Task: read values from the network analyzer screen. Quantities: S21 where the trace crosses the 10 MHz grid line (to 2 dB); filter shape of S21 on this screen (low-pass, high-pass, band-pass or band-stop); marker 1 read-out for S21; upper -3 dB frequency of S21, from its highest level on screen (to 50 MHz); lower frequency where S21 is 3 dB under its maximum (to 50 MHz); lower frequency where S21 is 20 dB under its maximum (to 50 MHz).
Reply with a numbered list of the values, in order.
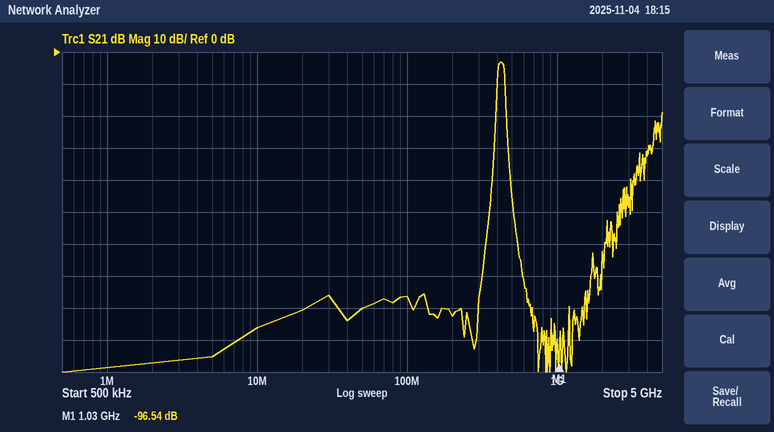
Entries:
1. -86 dB
2. band-pass
3. -96.54 dB
4. 450 MHz
5. 400 MHz
6. 400 MHz
